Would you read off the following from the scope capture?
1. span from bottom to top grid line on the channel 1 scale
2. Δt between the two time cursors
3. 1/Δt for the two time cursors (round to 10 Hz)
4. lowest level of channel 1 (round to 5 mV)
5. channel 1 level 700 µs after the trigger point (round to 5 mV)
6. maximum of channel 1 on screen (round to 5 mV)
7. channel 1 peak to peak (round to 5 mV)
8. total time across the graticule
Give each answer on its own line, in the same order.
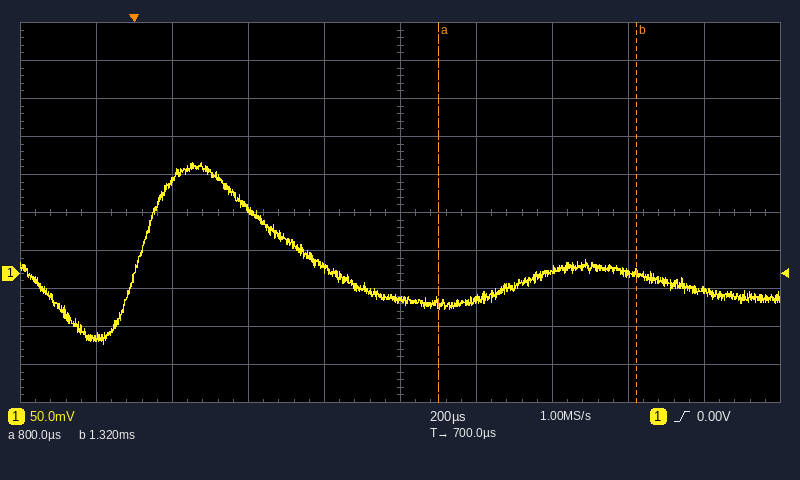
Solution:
500 mV
520 µs
1.92 kHz
-95 mV
-35 mV
145 mV
240 mV
2 ms
